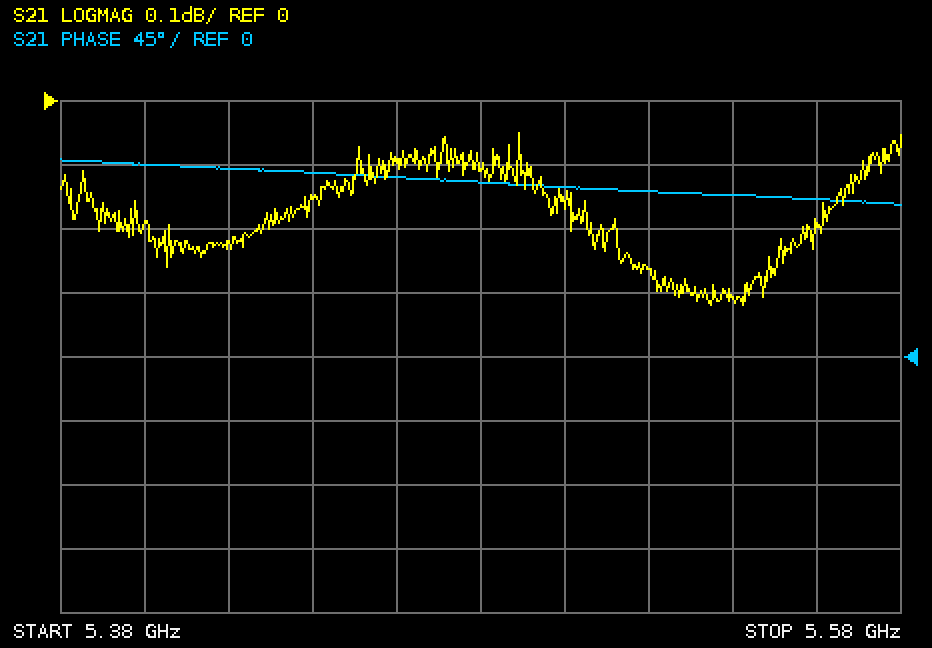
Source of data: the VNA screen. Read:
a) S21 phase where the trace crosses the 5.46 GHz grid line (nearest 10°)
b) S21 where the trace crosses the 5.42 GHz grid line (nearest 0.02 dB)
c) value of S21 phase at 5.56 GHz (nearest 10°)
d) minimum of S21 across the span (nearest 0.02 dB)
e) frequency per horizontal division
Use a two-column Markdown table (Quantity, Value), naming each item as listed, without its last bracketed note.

| Quantity | Value |
|---|---|
| S21 phase where the trace crosses the 5.46 GHz grid line | 130° |
| S21 where the trace crosses the 5.42 GHz grid line | -0.22 dB |
| value of S21 phase at 5.56 GHz | 110° |
| minimum of S21 across the span | -0.32 dB |
| frequency per horizontal division | 20 MHz |
